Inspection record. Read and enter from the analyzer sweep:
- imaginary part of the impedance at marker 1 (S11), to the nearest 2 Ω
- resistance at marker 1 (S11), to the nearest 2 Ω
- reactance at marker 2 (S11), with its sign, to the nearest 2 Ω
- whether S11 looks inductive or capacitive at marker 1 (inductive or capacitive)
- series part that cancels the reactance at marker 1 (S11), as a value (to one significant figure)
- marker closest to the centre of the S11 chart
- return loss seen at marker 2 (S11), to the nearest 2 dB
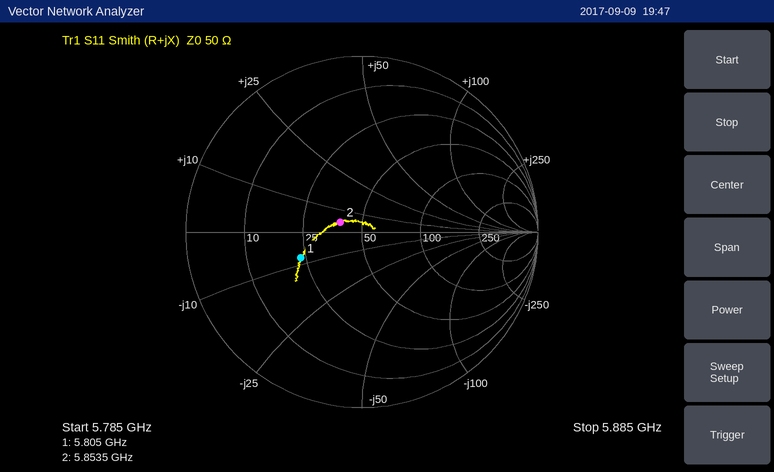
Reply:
-8 Ω
24 Ω
+4 Ω
capacitive
200 pH
marker 2
18 dB
